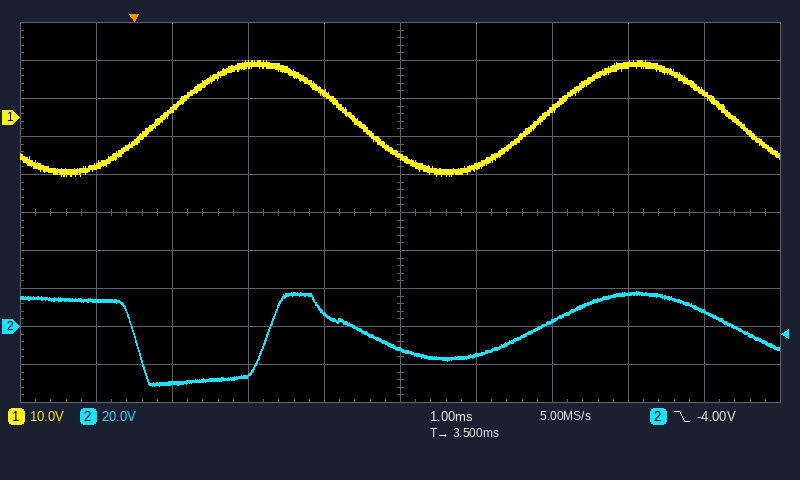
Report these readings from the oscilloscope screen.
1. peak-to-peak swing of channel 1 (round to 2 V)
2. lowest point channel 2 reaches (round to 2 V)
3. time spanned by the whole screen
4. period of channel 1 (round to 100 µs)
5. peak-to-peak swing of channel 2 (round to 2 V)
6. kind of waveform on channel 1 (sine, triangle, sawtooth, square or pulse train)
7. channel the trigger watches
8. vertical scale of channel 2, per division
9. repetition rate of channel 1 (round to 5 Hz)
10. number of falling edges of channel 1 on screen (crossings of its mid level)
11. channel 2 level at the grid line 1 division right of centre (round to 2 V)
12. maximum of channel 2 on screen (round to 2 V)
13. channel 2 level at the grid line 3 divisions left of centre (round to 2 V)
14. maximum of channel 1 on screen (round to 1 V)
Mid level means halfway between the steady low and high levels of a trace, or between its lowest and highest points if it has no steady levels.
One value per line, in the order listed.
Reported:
30 V
-32 V
10 ms
5.0 ms
50 V
sine
channel 2
20 V
200 Hz
2
-16 V
18 V
-30 V
15 V
